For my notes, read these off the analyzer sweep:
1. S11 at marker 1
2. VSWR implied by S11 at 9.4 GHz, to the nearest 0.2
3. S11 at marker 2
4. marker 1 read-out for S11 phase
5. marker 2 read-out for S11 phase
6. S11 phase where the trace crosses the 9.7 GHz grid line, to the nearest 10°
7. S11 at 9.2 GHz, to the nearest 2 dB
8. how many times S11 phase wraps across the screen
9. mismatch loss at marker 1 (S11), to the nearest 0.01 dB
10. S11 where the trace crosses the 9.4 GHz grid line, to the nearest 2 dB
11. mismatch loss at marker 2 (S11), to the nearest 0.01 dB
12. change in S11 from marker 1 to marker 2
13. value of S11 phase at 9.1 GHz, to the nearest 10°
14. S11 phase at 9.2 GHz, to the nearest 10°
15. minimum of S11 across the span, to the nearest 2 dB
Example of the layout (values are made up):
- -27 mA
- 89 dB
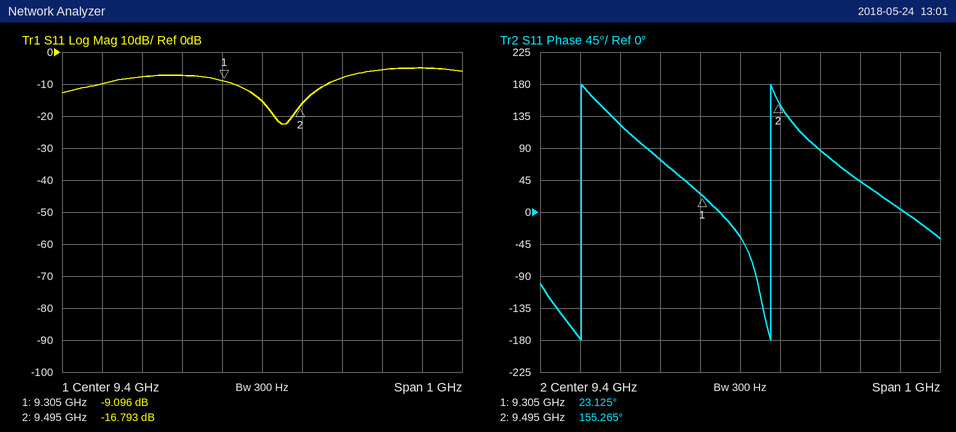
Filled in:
- -9.096 dB
- 1.4
- -16.793 dB
- 23.125°
- 155.265°
- 40°
- -8 dB
- 2
- 0.57 dB
- -16 dB
- 0.09 dB
- -7.697 dB
- 120°
- 70°
- -22 dB
